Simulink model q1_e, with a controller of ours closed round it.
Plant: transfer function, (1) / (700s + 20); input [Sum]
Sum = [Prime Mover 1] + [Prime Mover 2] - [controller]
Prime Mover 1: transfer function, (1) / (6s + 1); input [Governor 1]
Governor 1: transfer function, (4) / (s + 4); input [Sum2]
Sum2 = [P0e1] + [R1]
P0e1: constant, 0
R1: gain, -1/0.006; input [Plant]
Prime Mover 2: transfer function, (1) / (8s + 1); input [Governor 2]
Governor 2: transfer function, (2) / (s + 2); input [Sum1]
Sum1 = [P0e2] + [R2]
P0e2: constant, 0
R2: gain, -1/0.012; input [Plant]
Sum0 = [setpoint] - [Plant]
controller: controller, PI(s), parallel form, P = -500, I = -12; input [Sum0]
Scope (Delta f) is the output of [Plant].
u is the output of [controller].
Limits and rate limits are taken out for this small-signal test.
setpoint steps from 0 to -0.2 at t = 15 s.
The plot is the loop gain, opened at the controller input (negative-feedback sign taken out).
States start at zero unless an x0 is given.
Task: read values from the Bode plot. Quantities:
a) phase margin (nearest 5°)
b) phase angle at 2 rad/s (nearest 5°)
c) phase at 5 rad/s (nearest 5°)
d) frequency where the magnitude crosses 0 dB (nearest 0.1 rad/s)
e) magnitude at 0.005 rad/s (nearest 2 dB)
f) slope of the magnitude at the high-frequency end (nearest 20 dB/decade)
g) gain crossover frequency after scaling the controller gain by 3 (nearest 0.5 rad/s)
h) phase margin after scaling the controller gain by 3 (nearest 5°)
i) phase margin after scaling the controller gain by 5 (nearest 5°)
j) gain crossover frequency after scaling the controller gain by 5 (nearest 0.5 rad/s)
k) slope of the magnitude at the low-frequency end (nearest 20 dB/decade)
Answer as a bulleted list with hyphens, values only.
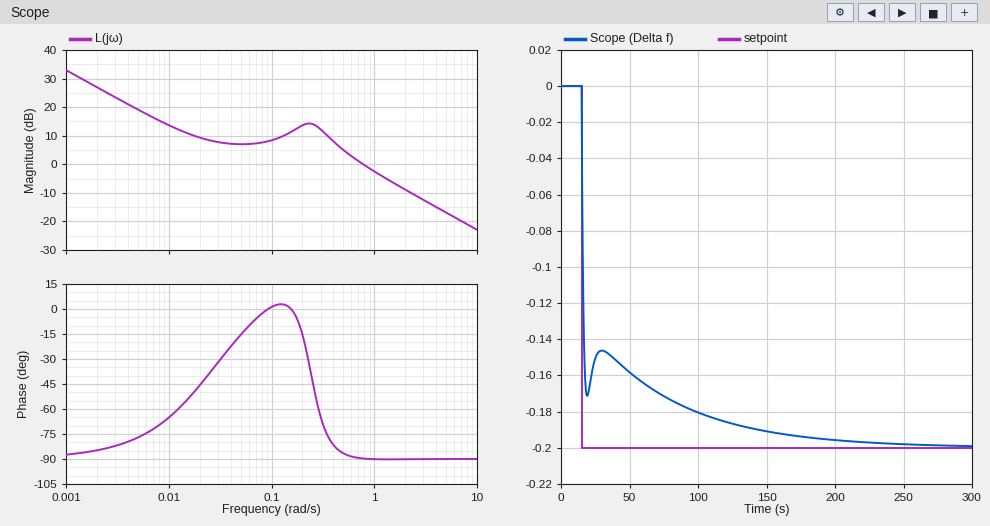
- 90°
- -90°
- -90°
- 0.8 rad/s
- 20 dB
- -20 dB/decade
- 2.0 rad/s
- 90°
- 90°
- 3.5 rad/s
- -20 dB/decade
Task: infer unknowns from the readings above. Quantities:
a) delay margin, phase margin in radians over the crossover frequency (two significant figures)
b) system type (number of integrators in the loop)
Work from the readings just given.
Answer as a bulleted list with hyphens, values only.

- 2.0 s
- 1
